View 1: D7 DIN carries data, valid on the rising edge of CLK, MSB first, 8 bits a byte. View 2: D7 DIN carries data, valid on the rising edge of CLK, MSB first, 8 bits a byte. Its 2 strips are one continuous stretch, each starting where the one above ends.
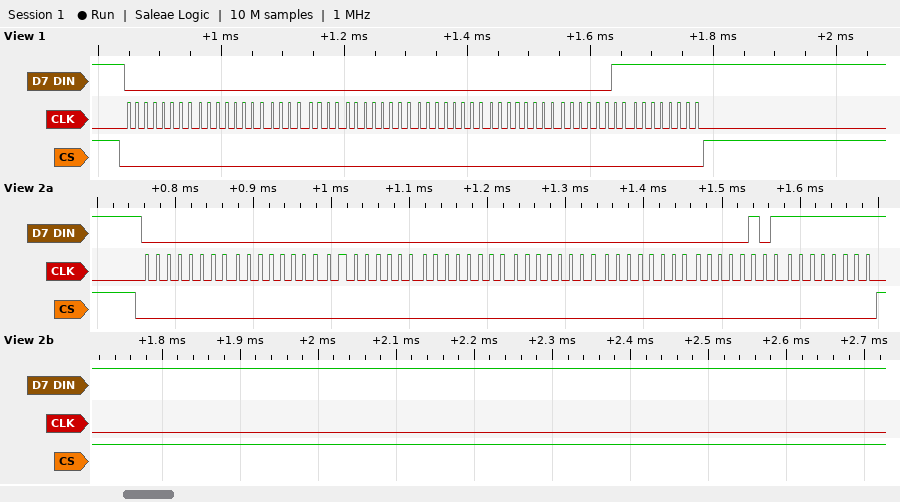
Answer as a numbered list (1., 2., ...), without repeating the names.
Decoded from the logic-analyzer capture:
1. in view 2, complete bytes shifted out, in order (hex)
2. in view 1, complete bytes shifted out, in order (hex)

1. 00 00 00 00 00 00 05 FF
2. 0x00 0x00 0x00 0x00 0x00 0x00 0x03 0xFF
